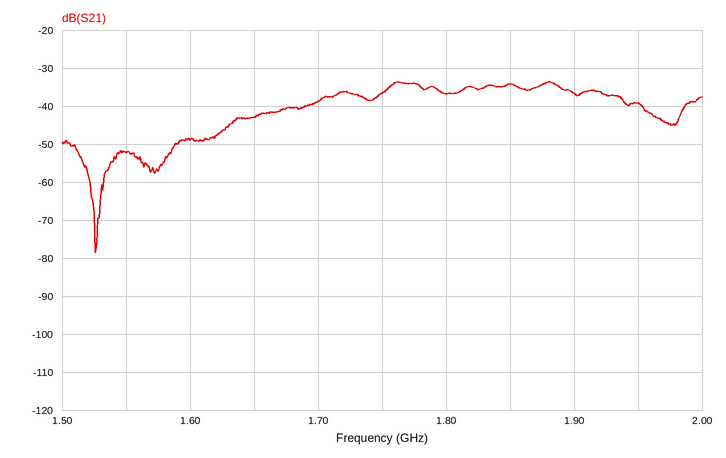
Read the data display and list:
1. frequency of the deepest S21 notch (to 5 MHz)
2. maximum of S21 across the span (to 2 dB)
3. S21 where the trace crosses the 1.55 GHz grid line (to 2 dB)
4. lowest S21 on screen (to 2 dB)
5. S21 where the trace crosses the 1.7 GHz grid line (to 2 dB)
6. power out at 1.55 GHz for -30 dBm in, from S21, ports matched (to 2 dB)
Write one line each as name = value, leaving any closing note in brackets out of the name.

frequency of the deepest S21 notch = 1.525 GHz
maximum of S21 across the span = -34 dB
S21 where the trace crosses the 1.55 GHz grid line = -52 dB
lowest S21 on screen = -78 dB
S21 where the trace crosses the 1.7 GHz grid line = -38 dB
power out at 1.55 GHz for -30 dBm in, from S21, ports matched = -82 dBm
